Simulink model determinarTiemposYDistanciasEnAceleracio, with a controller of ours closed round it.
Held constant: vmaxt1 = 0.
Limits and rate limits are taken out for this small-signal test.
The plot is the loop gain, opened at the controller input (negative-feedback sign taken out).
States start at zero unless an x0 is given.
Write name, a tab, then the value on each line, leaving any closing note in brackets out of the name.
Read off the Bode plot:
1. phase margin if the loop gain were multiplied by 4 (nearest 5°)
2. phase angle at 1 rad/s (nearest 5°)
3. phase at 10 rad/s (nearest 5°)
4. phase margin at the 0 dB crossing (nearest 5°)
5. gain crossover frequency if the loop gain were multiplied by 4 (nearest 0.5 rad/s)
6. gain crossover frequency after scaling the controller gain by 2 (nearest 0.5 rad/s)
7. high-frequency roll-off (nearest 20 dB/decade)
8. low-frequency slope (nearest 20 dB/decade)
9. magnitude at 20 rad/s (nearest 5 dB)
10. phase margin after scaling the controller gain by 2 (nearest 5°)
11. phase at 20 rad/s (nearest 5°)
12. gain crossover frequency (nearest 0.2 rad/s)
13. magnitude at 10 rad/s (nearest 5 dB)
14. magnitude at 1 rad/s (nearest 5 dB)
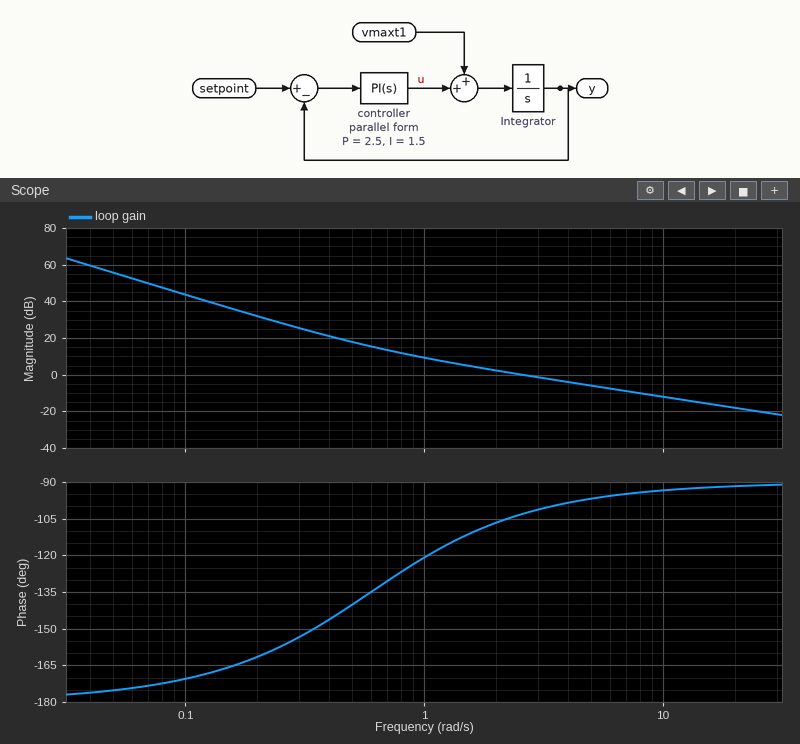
phase margin if the loop gain were multiplied by 4	85°
phase angle at 1 rad/s	-120°
phase at 10 rad/s	-95°
phase margin at the 0 dB crossing	75°
gain crossover frequency if the loop gain were multiplied by 4	10.0 rad/s
gain crossover frequency after scaling the controller gain by 2	5.0 rad/s
high-frequency roll-off	-20 dB/decade
low-frequency slope	-40 dB/decade
magnitude at 20 rad/s	-20 dB
phase margin after scaling the controller gain by 2	85°
phase at 20 rad/s	-90°
gain crossover frequency	2.6 rad/s
magnitude at 10 rad/s	-10 dB
magnitude at 1 rad/s	10 dB
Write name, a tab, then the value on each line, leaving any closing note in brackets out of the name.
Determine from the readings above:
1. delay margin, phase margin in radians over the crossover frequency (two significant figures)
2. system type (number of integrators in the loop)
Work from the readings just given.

delay margin, phase margin in radians over the crossover frequency	0.50 s
system type	2
